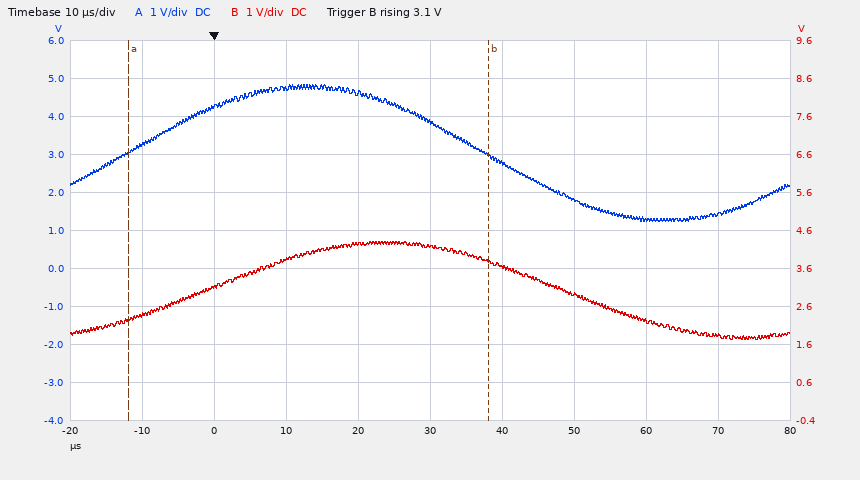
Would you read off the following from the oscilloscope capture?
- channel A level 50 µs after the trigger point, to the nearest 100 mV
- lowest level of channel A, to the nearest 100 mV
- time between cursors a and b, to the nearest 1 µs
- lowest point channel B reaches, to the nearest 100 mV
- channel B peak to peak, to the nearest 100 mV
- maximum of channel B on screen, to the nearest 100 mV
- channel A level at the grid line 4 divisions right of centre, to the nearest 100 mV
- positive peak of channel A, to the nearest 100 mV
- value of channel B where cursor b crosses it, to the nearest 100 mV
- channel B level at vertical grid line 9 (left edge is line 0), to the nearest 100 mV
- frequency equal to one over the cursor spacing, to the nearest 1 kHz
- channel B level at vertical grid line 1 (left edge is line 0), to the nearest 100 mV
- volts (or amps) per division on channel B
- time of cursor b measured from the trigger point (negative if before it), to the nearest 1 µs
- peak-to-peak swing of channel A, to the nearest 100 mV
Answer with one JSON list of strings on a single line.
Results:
["1.8 V", "1.2 V", "50 µs", "1.7 V", "2.6 V", "4.3 V", "1.4 V", "4.8 V", "3.8 V", "1.8 V", "20 kHz", "2.4 V", "1 V", "+38 µs", "3.6 V"]
